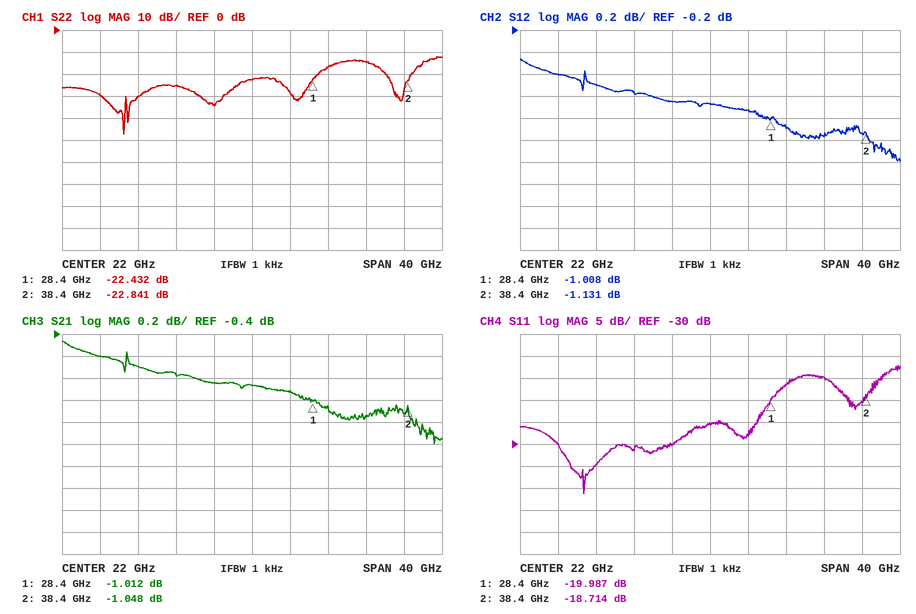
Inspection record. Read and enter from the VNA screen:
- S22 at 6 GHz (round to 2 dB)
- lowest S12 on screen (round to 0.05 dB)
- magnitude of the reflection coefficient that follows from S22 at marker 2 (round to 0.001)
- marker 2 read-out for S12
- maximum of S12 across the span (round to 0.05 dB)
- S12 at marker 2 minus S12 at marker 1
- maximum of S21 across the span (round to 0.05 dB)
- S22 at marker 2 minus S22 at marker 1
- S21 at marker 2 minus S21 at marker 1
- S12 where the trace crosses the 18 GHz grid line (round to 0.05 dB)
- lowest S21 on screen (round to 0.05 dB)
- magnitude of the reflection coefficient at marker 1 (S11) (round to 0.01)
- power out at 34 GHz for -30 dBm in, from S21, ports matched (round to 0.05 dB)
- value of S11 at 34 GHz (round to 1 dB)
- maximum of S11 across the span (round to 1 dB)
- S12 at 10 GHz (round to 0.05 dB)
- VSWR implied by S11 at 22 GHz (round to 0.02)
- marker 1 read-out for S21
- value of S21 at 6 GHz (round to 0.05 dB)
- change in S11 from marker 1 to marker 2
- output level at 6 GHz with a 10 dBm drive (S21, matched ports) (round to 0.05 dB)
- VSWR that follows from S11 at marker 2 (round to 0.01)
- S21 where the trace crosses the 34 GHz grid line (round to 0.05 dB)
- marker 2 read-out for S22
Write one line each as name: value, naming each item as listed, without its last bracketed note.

S22 at 6 GHz: -30 dB
lowest S12 on screen: -1.40 dB
magnitude of the reflection coefficient that follows from S22 at marker 2: 0.072
marker 2 read-out for S12: -1.131 dB
maximum of S12 across the span: -0.45 dB
S12 at marker 2 minus S12 at marker 1: -0.123 dB
maximum of S21 across the span: -0.45 dB
S22 at marker 2 minus S22 at marker 1: -0.409 dB
S21 at marker 2 minus S21 at marker 1: -0.036 dB
S12 where the trace crosses the 18 GHz grid line: -0.85 dB
lowest S21 on screen: -1.40 dB
magnitude of the reflection coefficient at marker 1 (S11): 0.10
power out at 34 GHz for -30 dBm in, from S21, ports matched: -31.15 dBm
value of S11 at 34 GHz: -15 dB
maximum of S11 across the span: -12 dB
S12 at 10 GHz: -0.70 dB
VSWR implied by S11 at 22 GHz: 1.12
marker 1 read-out for S21: -1.012 dB
value of S21 at 6 GHz: -0.60 dB
change in S11 from marker 1 to marker 2: 1.273 dB
output level at 6 GHz with a 10 dBm drive (S21, matched ports): 9.40 dBm
VSWR that follows from S11 at marker 2: 1.26
S21 where the trace crosses the 34 GHz grid line: -1.15 dB
marker 2 read-out for S22: -22.841 dB
